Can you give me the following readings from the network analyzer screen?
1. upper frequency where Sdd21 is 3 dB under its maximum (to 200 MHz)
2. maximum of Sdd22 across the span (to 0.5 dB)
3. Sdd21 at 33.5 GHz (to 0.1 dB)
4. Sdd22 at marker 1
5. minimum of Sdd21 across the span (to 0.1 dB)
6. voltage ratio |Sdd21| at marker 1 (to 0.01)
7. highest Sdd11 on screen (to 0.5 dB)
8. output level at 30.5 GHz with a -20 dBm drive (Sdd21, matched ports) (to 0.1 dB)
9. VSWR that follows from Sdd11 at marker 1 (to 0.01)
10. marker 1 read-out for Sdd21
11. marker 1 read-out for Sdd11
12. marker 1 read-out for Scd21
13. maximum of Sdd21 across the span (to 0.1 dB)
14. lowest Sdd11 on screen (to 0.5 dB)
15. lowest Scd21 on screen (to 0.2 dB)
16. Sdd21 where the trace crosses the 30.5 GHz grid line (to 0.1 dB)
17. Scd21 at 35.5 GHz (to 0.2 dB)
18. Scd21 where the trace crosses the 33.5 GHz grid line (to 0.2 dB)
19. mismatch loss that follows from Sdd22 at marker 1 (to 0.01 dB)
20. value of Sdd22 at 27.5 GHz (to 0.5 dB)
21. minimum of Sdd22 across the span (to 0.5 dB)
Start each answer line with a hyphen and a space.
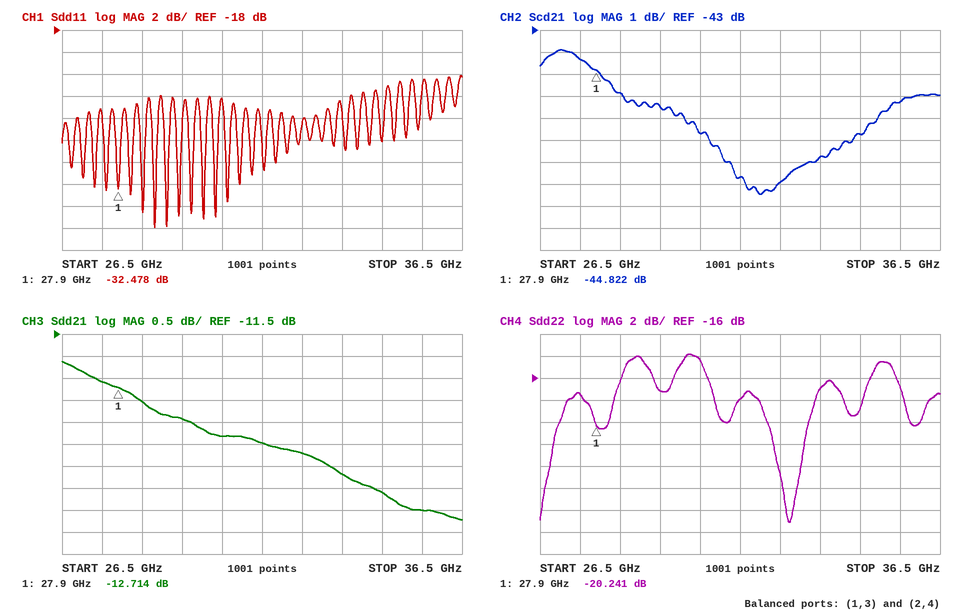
- 34.6 GHz
- -14.0 dB
- -14.7 dB
- -20.241 dB
- -15.7 dB
- 0.23
- -22.0 dB
- -33.8 dBm
- 1.05
- -12.714 dB
- -32.478 dB
- -44.822 dB
- -12.1 dB
- -36.0 dB
- -50.4 dB
- -13.8 dB
- -46.2 dB
- -48.8 dB
- 0.04 dB
- -17.5 dB
- -29.0 dB
